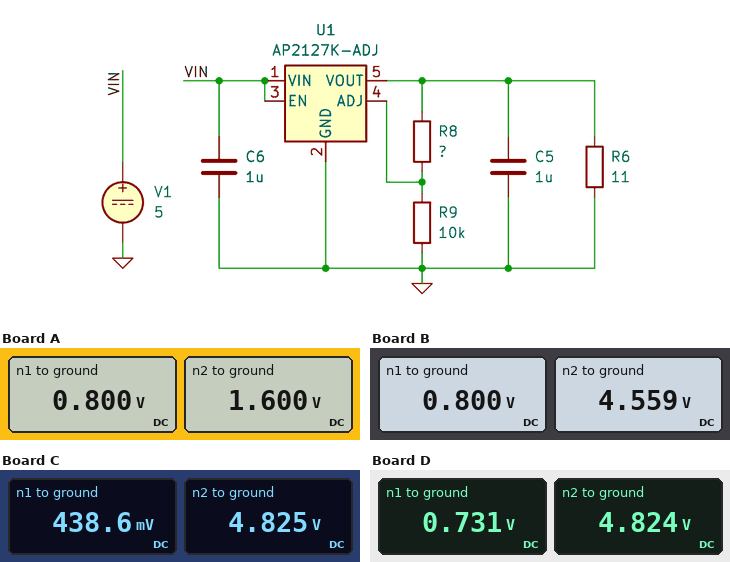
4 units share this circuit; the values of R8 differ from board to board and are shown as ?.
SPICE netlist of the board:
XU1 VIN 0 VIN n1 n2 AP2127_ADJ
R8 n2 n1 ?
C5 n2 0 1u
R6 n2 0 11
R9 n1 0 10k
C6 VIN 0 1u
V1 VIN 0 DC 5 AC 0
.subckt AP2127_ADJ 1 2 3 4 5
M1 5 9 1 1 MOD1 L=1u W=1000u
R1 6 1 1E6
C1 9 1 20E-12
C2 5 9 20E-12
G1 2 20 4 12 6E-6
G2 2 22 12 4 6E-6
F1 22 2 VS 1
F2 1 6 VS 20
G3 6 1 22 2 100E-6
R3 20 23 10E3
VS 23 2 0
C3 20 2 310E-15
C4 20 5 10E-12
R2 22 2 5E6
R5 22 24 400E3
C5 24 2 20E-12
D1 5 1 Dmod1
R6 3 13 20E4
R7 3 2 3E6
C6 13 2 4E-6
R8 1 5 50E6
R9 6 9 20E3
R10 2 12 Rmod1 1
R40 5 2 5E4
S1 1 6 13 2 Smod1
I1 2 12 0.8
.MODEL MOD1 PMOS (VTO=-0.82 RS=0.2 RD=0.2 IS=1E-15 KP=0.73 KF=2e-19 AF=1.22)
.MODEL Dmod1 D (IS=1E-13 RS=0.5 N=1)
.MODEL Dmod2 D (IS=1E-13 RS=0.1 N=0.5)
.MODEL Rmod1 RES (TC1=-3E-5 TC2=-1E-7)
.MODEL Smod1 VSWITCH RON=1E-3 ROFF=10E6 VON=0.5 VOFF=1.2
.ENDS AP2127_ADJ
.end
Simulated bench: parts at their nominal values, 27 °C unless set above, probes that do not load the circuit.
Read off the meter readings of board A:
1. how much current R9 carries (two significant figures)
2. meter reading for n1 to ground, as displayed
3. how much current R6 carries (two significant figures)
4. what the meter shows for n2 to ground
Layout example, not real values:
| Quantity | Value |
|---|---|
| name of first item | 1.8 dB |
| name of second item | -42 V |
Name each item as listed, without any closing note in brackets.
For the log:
| Quantity | Value |
|---|---|
| how much current R9 carries | 80 µA |
| meter reading for n1 to ground, as displayed | 0.800 V |
| how much current R6 carries | 150 mA |
| what the meter shows for n2 to ground | 1.600 V |
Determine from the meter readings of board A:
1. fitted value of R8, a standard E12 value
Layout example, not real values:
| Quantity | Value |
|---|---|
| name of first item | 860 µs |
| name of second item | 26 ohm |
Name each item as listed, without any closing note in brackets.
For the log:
| Quantity | Value |
|---|---|
| fitted value of R8, a standard E12 value | 10 kΩ |
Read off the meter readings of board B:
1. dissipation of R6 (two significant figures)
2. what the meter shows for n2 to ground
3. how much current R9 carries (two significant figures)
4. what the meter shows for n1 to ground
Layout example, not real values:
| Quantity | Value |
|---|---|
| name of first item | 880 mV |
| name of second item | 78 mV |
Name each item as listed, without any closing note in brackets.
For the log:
| Quantity | Value |
|---|---|
| dissipation of R6 | 1.9 W |
| what the meter shows for n2 to ground | 4.559 V |
| how much current R9 carries | 80 µA |
| what the meter shows for n1 to ground | 0.800 V |
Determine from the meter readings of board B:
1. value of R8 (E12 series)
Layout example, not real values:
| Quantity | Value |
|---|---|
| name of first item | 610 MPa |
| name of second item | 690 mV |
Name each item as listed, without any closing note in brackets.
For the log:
| Quantity | Value |
|---|---|
| value of R8 | 47 kΩ |
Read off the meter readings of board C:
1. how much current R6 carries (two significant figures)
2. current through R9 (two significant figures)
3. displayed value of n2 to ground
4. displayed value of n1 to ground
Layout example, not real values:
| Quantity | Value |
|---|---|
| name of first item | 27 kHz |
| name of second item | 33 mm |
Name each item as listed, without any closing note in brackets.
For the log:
| Quantity | Value |
|---|---|
| how much current R6 carries | 440 mA |
| current through R9 | 44 µA |
| displayed value of n2 to ground | 4.825 V |
| displayed value of n1 to ground | 438.6 mV |
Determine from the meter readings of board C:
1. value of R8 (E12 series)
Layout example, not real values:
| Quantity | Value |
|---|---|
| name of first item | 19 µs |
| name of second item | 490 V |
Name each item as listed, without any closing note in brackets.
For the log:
| Quantity | Value |
|---|---|
| value of R8 | 100 kΩ |
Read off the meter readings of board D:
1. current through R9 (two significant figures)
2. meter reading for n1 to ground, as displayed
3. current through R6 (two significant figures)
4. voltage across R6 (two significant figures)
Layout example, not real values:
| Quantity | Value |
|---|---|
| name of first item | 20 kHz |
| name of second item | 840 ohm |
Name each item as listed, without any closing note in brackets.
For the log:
| Quantity | Value |
|---|---|
| current through R9 | 73 µA |
| meter reading for n1 to ground, as displayed | 0.731 V |
| current through R6 | 440 mA |
| voltage across R6 | 4.8 V |
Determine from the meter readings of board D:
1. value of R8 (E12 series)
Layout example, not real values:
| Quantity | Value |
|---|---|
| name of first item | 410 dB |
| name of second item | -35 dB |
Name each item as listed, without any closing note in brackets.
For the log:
| Quantity | Value |
|---|---|
| value of R8 | 56 kΩ |
